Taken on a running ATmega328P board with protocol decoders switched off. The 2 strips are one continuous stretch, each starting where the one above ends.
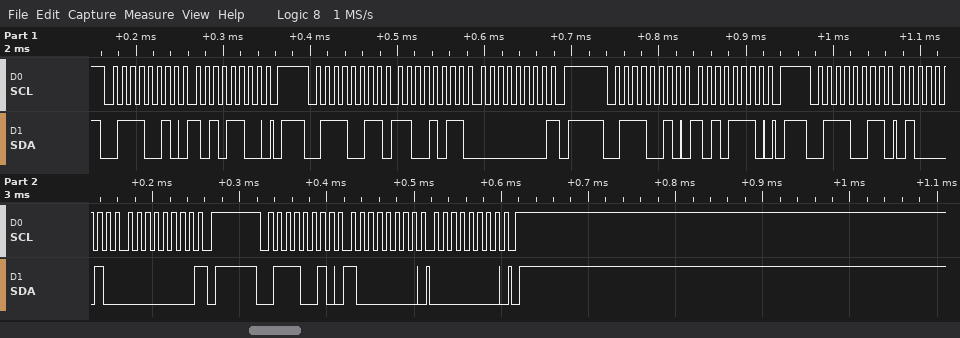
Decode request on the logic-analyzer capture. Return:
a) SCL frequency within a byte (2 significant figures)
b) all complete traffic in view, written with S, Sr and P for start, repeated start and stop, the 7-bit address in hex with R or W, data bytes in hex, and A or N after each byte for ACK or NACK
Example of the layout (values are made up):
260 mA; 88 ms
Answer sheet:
100 kHz; S 39W A AC A P S 39R A CB A 00 N P S 39W A AE A P S 39R A 42 A 00 N P S 39W A 80 A 00 A P
